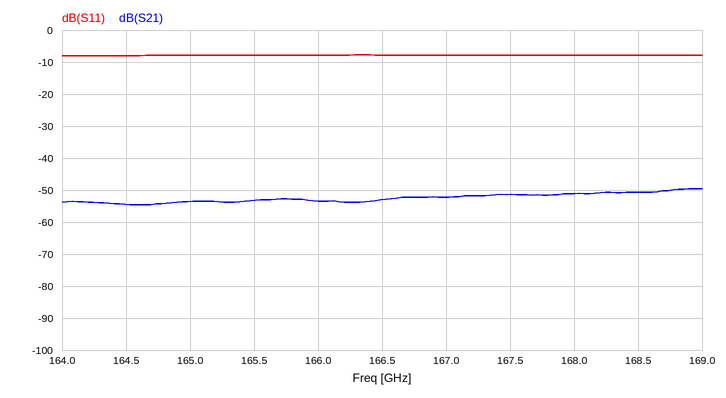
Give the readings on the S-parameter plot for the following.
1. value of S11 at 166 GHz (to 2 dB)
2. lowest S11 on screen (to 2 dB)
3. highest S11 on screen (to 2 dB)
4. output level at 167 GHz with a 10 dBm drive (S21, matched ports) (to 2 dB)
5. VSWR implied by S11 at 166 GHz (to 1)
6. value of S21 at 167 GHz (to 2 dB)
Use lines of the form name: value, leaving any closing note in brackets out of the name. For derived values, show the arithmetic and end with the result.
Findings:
value of S11 at 166 GHz: -8 dB
lowest S11 on screen: -8 dB
highest S11 on screen: -8 dB
output level at 167 GHz with a 10 dBm drive (S21, matched ports): 10 dBm + (-52 dB) = -42 dBm
VSWR implied by S11 at 166 GHz: |Γ| = 10^(-8/20) = 0.3981; VSWR = (1 + 0.3981)/(1 − 0.3981) ≈ 2
value of S21 at 167 GHz: -52 dB
